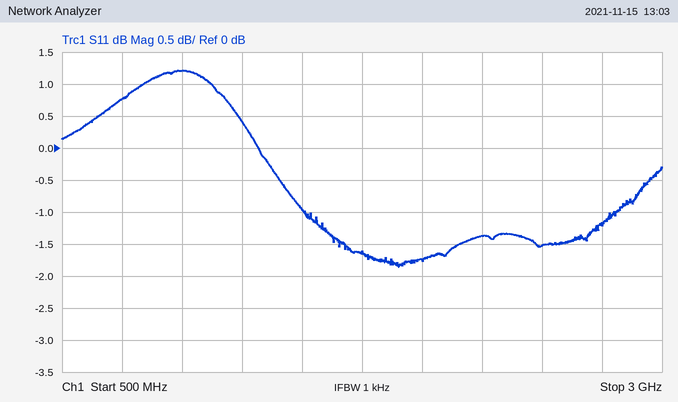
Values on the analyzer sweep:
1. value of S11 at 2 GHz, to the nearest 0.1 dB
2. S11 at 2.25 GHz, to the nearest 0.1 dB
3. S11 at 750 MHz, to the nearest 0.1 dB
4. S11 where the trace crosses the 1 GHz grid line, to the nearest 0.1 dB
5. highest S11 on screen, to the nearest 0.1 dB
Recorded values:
-1.7 dB
-1.4 dB
0.8 dB
1.2 dB
1.2 dB
